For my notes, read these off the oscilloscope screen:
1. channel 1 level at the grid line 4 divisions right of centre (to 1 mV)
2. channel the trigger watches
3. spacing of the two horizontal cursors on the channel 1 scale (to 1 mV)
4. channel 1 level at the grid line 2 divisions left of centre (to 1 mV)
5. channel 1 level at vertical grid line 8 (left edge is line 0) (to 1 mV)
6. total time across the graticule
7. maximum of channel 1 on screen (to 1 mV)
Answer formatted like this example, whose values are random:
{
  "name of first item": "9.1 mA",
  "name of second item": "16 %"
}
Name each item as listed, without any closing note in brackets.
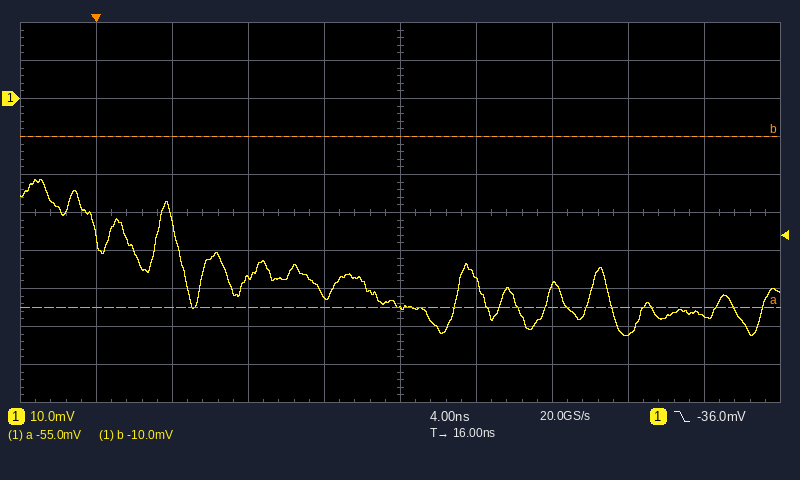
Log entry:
{
  "channel 1 level at the grid line 4 divisions right of centre": "-57 mV",
  "channel the trigger watches": "channel 1",
  "spacing of the two horizontal cursors on the channel 1 scale": "45 mV",
  "channel 1 level at the grid line 2 divisions left of centre": "-47 mV",
  "channel 1 level at vertical grid line 8 (left edge is line 0)": "-62 mV",
  "total time across the graticule": "40 ns",
  "maximum of channel 1 on screen": "-21 mV"
}
